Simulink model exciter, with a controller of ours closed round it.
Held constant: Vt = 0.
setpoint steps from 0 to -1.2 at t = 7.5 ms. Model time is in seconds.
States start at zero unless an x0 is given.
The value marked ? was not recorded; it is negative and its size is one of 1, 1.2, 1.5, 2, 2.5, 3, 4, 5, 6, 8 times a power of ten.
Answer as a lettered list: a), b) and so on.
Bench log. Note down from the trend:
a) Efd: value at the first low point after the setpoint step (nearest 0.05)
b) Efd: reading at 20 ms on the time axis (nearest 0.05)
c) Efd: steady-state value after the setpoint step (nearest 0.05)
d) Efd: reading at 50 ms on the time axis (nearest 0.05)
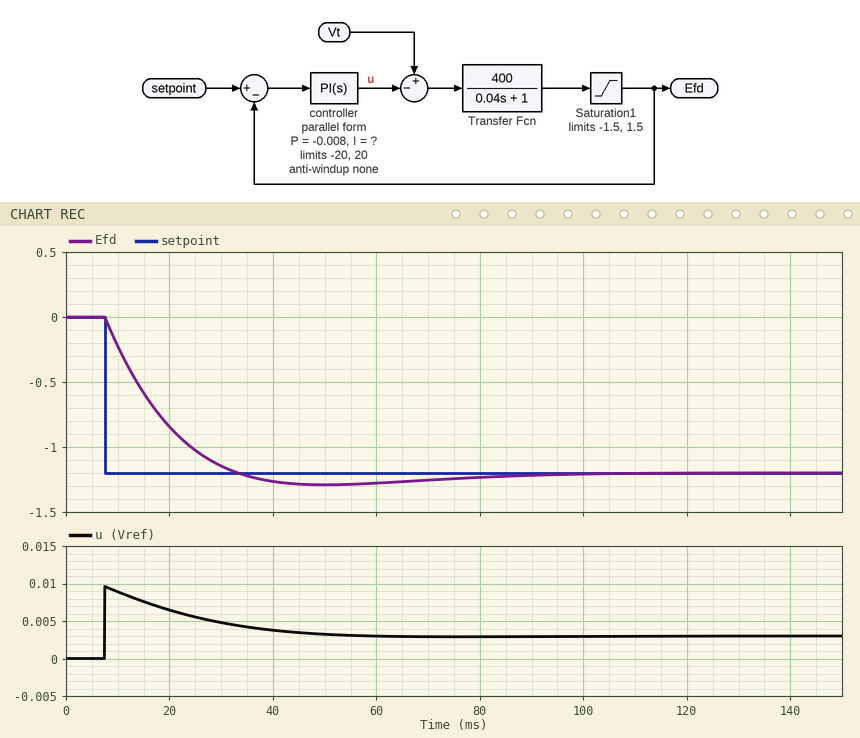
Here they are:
a) -1.30
b) -0.85
c) -1.20
d) -1.30
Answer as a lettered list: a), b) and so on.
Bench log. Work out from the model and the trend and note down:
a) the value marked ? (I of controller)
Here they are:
a) -0.4
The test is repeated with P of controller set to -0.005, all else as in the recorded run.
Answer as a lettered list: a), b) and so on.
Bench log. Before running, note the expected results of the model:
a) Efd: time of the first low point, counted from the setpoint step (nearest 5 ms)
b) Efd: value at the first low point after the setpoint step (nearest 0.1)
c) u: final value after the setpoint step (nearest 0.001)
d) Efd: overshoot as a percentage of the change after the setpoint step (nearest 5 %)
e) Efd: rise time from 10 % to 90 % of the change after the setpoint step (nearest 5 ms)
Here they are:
a) 45 ms
b) -1.4
c) 0.003
d) 15 %
e) 20 ms
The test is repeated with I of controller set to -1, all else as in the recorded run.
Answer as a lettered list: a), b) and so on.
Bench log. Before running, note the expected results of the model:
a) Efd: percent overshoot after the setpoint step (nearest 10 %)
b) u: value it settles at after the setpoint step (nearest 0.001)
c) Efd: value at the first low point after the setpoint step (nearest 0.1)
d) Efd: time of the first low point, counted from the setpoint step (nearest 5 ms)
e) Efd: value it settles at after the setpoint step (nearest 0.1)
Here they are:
a) 20 %
b) 0.003
c) -1.5
d) 25 ms
e) -1.2
